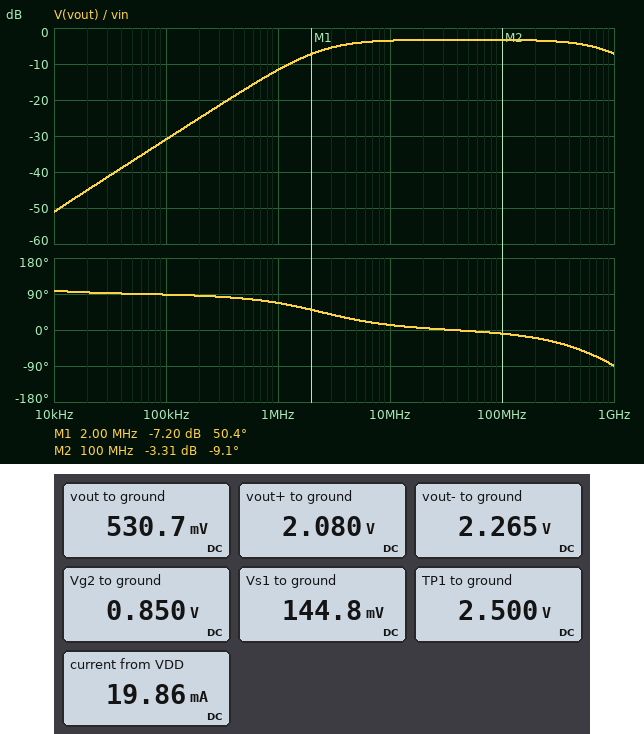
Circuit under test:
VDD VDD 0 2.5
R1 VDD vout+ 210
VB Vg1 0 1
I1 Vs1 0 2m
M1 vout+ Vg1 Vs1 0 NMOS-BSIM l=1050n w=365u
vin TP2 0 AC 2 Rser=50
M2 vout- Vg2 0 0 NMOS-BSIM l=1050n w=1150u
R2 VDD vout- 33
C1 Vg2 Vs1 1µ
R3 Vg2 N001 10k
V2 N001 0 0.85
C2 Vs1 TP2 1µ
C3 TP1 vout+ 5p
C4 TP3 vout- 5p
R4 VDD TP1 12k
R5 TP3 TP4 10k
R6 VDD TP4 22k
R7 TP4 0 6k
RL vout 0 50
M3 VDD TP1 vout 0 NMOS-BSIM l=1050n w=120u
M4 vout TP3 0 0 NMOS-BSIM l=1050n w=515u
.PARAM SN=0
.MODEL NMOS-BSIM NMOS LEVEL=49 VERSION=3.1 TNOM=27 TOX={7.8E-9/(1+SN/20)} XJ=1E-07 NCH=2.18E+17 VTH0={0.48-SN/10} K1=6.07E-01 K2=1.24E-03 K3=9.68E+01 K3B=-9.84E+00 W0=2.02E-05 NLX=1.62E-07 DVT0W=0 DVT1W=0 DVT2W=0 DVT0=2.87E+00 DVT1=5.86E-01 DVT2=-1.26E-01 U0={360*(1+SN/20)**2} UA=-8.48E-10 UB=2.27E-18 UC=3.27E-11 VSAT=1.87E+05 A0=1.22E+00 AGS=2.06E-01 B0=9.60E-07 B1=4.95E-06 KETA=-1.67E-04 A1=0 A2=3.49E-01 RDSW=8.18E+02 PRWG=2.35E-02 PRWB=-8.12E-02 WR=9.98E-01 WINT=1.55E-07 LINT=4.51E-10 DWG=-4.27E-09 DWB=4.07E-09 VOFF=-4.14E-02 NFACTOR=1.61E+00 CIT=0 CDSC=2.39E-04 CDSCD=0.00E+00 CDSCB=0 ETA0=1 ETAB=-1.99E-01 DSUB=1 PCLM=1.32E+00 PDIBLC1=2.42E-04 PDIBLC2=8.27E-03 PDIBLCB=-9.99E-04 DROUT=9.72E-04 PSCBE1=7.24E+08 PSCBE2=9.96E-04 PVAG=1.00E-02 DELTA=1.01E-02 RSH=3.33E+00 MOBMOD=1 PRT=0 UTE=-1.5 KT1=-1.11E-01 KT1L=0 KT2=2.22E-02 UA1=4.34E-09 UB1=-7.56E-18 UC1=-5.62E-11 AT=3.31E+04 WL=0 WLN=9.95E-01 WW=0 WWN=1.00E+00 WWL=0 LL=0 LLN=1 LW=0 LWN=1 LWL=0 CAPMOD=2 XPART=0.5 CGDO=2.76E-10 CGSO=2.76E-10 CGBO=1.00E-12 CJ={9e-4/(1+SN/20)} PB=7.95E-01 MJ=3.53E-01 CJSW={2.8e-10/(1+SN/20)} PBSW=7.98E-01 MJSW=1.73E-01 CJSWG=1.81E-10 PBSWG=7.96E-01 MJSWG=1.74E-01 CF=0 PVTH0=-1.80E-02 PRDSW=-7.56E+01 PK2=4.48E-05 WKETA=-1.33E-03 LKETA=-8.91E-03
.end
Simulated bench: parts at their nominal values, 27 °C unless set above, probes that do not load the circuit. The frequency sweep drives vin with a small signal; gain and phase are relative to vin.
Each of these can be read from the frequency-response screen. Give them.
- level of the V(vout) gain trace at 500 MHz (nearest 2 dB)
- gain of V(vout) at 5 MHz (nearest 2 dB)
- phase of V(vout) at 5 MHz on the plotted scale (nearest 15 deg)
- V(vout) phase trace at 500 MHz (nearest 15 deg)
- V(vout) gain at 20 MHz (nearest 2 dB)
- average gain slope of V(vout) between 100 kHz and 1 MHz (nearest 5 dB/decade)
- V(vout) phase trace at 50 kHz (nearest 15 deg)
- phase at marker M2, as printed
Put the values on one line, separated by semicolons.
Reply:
-4 dB; -4 dB; 30 deg; -45 deg; -4 dB; 20 dB/decade; 90 deg; -9.1 deg
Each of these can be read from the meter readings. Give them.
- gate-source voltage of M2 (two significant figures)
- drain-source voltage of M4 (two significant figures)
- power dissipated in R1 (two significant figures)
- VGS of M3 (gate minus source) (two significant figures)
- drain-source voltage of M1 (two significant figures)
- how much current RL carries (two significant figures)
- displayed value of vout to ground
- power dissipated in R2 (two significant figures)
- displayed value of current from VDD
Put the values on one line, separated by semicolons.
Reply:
850 mV; 530 mV; 840 µW; 2.0 V; 1.9 V; 11 mA; 530.7 mV; 1.7 mW; 19.86 mA
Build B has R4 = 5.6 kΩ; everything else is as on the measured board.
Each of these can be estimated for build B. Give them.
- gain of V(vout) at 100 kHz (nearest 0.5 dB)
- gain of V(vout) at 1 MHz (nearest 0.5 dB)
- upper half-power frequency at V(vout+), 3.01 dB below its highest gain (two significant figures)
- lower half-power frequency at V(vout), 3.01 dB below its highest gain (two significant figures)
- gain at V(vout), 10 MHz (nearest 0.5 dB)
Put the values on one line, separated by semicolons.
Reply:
-37.5 dB; -17.5 dB; 800 MHz; 5.1 MHz; -4.5 dB
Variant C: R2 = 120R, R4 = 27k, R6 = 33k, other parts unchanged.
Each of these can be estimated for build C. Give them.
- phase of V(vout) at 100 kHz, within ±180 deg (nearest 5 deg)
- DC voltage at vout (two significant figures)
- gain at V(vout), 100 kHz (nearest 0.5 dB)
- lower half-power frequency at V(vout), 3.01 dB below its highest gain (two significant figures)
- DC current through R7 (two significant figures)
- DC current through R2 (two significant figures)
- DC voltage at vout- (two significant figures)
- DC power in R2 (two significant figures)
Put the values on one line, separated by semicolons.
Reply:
85 deg; 530 mV; -24.0 dB; 1.1 MHz; 64 µA; 7.0 mA; 1.7 V; 5.8 mW
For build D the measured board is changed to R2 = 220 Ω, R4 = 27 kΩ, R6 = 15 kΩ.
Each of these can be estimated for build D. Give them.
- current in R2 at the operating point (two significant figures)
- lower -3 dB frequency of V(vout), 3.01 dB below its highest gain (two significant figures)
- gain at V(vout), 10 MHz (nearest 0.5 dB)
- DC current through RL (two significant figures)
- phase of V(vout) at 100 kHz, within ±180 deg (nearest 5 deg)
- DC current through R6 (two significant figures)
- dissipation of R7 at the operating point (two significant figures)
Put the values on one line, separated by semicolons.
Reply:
6.8 mA; 1.4 MHz; 4.5 dB; 10 mA; 85 deg; 120 µA; 85 µW
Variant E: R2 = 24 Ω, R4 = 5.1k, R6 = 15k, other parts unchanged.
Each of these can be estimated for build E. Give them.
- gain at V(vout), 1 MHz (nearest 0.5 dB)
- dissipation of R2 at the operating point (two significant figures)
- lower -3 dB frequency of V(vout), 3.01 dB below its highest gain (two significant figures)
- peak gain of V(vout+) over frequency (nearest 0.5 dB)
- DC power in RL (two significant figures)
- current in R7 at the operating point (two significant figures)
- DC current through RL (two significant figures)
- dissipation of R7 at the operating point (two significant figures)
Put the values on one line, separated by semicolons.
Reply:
-15.0 dB; 1.2 mW; 5.2 MHz; 6.0 dB; 5.1 mW; 120 µA; 10 mA; 85 µW
